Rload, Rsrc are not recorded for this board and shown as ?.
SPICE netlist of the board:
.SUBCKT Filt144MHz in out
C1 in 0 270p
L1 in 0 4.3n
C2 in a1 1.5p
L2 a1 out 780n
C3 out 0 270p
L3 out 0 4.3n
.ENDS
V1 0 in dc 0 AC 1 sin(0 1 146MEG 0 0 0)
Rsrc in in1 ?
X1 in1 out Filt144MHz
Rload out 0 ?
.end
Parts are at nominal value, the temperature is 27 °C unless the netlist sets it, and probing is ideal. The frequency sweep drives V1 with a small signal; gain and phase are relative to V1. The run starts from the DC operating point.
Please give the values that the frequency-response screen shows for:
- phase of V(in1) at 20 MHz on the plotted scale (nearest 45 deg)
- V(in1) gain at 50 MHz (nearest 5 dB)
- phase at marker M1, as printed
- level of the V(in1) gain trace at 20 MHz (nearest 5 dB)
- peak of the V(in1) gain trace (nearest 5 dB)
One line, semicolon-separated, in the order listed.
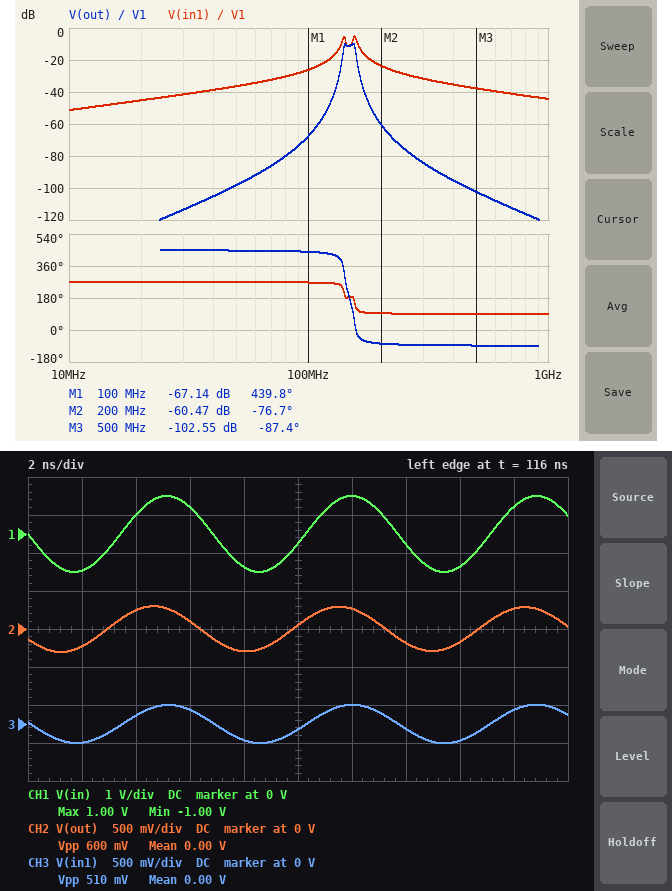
270 deg; -35 dB; 439.8 deg; -45 dB; -5 dB
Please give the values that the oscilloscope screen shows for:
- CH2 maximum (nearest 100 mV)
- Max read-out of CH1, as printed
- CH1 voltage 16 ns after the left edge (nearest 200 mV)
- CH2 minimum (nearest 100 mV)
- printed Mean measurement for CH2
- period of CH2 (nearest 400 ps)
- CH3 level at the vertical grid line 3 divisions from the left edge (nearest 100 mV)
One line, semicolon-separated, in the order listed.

300 mV; 1.00 V; -800 mV; -300 mV; 0.00 V; 6.8 ns; 200 mV
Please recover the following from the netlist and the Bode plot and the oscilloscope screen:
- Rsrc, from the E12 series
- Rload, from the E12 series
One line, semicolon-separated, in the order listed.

100 Ω; 39 Ω
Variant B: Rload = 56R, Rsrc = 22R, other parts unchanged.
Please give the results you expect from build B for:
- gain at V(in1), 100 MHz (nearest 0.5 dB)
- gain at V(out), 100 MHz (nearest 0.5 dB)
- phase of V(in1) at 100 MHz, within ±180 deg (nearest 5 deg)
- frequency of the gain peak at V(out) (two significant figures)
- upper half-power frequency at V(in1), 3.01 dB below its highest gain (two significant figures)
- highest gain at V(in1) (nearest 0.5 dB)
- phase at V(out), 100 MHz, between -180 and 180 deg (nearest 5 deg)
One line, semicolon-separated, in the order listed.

-13.0 dB; -54.0 dB; -105 deg; 140 MHz; 170 MHz; -1.0 dB; 70 deg
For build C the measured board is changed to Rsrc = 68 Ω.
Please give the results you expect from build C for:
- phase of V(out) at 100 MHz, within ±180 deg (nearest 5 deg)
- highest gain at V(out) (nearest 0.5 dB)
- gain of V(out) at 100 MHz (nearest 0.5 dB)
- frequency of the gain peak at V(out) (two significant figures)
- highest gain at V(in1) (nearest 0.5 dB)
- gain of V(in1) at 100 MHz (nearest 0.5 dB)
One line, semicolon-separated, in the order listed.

80 deg; -8.5 dB; -64.0 dB; 140 MHz; -3.5 dB; -22.5 dB
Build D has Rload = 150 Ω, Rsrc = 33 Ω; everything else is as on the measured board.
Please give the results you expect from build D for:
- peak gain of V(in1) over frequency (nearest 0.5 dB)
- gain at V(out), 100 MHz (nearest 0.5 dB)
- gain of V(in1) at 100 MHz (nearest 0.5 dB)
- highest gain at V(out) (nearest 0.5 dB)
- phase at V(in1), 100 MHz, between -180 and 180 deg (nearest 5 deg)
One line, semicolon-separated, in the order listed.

-1.0 dB; -57.5 dB; -16.5 dB; 0.5 dB; -100 deg
